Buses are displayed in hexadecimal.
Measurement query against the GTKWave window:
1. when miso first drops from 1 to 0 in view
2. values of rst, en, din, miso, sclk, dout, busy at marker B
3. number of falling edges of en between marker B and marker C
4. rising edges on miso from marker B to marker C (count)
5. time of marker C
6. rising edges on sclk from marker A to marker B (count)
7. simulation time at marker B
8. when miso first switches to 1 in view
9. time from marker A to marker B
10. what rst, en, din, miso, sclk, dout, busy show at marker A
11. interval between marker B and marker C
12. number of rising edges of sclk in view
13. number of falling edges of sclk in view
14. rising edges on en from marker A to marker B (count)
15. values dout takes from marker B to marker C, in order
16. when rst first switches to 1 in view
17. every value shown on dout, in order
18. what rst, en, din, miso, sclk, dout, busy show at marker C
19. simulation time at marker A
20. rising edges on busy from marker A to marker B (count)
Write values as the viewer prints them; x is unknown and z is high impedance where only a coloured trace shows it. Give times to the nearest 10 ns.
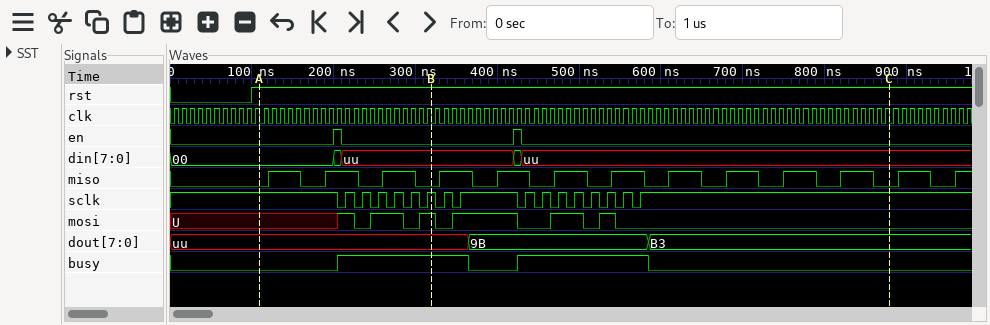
160 ns
rst=1, en=0, din=uu, miso=0, sclk=1, dout=uu, busy=1
1
8
880 ns
6
320 ns
120 ns
210 ns
rst=1, en=0, din=00, miso=0, sclk=1, dout=uu, busy=0
560 ns
16
16
1
uu, 9B, B3
100 ns
uu, 9B, B3
rst=1, en=0, din=uu, miso=0, sclk=1, dout=B3, busy=0
110 ns
1
